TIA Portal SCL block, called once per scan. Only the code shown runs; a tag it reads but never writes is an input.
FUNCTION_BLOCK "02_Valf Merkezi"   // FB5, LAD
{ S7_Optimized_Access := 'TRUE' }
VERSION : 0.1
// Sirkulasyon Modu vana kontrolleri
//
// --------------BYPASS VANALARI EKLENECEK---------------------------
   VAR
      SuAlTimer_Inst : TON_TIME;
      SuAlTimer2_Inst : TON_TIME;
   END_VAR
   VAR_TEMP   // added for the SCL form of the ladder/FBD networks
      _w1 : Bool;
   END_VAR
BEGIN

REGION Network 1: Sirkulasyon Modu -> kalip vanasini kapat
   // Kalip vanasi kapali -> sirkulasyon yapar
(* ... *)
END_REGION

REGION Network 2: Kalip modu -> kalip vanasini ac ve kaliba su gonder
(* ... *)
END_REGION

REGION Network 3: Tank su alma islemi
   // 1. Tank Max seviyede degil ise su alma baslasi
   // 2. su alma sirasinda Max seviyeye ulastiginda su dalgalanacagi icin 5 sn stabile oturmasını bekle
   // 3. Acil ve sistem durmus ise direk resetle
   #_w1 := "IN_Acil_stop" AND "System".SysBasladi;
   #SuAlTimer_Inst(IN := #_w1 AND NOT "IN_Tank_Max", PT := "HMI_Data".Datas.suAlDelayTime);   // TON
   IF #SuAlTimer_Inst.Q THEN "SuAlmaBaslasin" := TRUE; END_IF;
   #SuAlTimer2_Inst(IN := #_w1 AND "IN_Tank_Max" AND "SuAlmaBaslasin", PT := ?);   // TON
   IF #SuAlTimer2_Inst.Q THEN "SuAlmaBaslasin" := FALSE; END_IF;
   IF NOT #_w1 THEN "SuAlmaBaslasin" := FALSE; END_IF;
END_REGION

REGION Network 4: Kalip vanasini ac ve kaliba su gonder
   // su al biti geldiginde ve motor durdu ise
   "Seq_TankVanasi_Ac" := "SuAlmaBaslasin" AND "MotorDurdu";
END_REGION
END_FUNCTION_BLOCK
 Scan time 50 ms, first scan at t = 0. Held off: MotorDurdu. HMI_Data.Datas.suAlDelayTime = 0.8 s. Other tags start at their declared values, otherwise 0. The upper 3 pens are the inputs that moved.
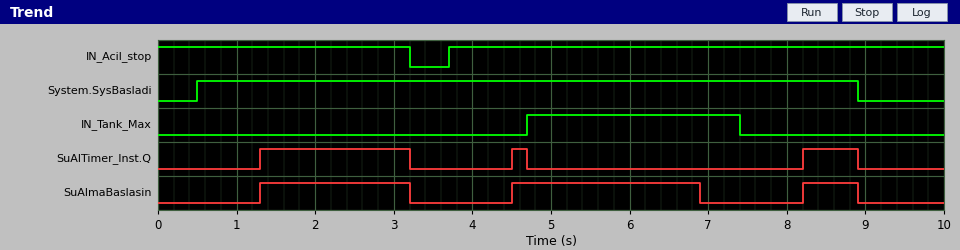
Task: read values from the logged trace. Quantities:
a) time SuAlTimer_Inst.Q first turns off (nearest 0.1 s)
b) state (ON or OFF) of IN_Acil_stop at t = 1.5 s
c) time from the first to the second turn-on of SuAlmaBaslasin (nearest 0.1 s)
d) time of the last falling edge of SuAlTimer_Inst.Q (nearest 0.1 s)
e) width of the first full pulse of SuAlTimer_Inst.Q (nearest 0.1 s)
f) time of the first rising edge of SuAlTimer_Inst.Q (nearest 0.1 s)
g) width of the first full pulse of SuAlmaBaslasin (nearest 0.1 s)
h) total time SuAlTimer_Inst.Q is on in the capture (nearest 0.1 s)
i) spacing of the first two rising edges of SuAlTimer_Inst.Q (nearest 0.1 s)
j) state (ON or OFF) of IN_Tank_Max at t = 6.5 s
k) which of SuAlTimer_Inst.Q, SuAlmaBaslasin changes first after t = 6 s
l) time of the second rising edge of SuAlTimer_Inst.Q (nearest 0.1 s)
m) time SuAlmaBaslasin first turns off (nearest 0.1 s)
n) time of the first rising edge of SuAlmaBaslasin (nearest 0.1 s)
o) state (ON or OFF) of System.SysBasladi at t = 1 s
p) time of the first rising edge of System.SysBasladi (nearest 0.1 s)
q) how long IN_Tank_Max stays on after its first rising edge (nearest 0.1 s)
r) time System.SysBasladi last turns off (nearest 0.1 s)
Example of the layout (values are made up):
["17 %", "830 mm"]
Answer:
["3.2 s", "ON", "3.2 s", "8.9 s", "1.9 s", "1.3 s", "1.9 s", "2.8 s", "3.2 s", "ON", "SuAlmaBaslasin", "4.5 s", "3.2 s", "1.3 s", "ON", "0.5 s", "2.7 s", "8.9 s"]
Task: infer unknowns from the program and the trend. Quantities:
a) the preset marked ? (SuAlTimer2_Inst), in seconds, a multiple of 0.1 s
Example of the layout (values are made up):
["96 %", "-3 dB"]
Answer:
["2.2 s"]
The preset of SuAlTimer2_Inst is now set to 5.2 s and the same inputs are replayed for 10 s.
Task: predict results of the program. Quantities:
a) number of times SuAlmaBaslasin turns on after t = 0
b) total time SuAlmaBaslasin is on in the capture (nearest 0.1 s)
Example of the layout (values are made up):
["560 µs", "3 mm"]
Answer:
["2", "6.3 s"]
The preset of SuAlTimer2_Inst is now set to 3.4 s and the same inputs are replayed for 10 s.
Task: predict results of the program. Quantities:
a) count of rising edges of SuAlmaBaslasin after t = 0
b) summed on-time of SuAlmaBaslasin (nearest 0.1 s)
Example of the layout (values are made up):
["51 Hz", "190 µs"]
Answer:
["2", "6.3 s"]
